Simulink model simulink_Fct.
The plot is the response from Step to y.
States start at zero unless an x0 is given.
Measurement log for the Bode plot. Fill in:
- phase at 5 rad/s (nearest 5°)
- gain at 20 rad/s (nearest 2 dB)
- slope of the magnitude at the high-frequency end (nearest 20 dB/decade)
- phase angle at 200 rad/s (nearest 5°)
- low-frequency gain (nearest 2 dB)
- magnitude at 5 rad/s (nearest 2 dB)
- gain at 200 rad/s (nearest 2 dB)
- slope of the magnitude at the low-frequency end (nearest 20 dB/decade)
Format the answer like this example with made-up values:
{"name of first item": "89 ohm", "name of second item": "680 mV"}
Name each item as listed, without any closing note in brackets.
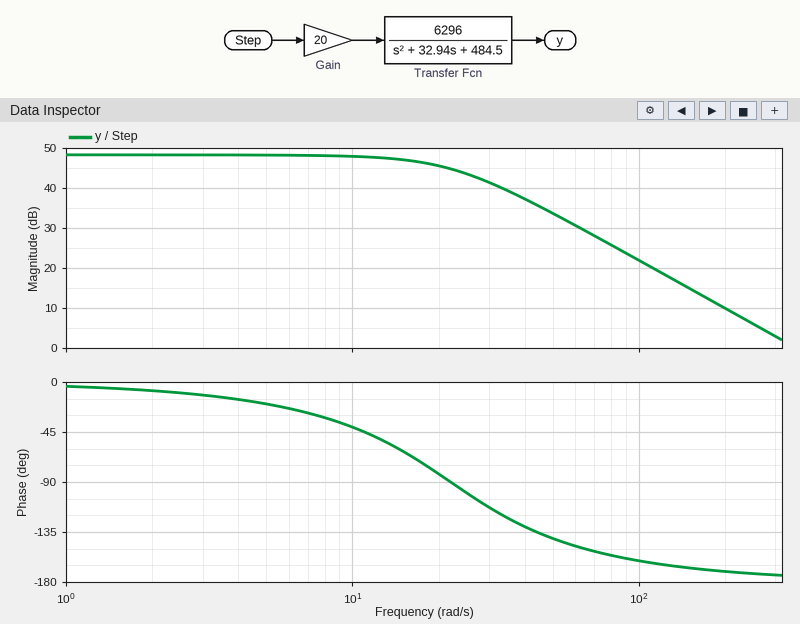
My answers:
{"phase at 5 rad/s": "-20°", "gain at 20 rad/s": "46 dB", "slope of the magnitude at the high-frequency end": "-40 dB/decade", "phase angle at 200 rad/s": "-170°", "low-frequency gain": "48 dB", "magnitude at 5 rad/s": "48 dB", "gain at 200 rad/s": "10 dB", "slope of the magnitude at the low-frequency end": "0 dB/decade"}
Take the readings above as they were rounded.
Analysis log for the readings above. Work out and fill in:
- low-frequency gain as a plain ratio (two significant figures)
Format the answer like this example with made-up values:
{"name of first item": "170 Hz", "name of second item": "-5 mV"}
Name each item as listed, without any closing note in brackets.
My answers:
{"low-frequency gain as a plain ratio": "250"}
